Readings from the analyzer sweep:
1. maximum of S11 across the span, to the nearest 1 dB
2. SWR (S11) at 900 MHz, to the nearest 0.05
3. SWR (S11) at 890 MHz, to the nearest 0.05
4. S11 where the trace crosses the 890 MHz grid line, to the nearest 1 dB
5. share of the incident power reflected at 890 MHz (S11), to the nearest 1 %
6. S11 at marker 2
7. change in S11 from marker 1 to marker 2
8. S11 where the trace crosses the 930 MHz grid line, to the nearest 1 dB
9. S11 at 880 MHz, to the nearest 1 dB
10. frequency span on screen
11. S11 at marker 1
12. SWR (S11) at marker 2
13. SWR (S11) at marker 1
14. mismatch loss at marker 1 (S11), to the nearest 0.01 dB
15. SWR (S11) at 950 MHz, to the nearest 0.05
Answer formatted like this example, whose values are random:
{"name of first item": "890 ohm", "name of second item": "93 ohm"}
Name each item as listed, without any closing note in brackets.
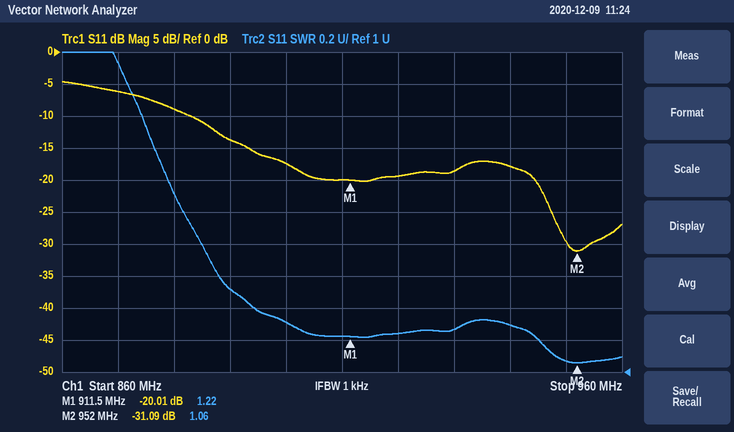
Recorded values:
{"maximum of S11 across the span, to the nearest 1 dB": "-5 dB", "SWR (S11) at 900 MHz, to the nearest 0.05": "1.30", "SWR (S11) at 890 MHz, to the nearest 0.05": "1.50", "S11 where the trace crosses the 890 MHz grid line, to the nearest 1 dB": "-14 dB", "share of the incident power reflected at 890 MHz (S11), to the nearest 1 %": "4 %", "S11 at marker 2": "-31.09 dB", "change in S11 from marker 1 to marker 2": "-11.08 dB", "S11 where the trace crosses the 930 MHz grid line, to the nearest 1 dB": "-19 dB", "S11 at 880 MHz, to the nearest 1 dB": "-9 dB", "frequency span on screen": "100 MHz", "S11 at marker 1": "-20.01 dB", "SWR (S11) at marker 2": "1.06", "SWR (S11) at marker 1": "1.22", "mismatch loss at marker 1 (S11), to the nearest 0.01 dB": "0.04 dB", "SWR (S11) at 950 MHz, to the nearest 0.05": "1.05"}
